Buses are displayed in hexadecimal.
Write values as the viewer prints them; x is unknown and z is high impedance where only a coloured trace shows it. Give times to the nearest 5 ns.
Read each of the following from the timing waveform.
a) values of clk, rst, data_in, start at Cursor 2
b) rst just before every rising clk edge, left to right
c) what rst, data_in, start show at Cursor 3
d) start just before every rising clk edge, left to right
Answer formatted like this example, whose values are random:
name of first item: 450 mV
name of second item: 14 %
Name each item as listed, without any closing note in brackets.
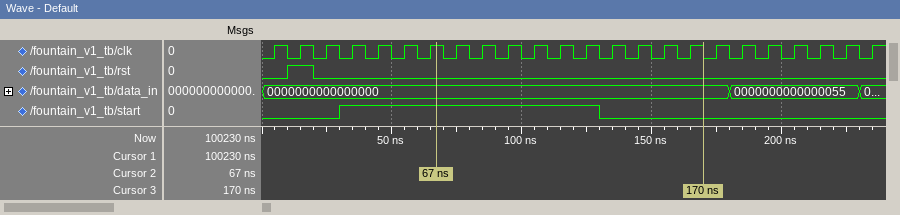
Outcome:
values of clk, rst, data_in, start at Cursor 2: clk=1, rst=0, data_in=0000000000000000, start=1
rst just before every rising clk edge, left to right: 0 1 0 0 0 0 0 0 0 0 0 0 0 0 0 0 0 0 0 0 0 0 0 0
what rst, data_in, start show at Cursor 3: rst=0, data_in=0000000000000000, start=0
start just before every rising clk edge, left to right: 0 0 0 1 1 1 1 1 1 1 1 1 1 0 0 0 0 0 0 0 0 0 0 0
